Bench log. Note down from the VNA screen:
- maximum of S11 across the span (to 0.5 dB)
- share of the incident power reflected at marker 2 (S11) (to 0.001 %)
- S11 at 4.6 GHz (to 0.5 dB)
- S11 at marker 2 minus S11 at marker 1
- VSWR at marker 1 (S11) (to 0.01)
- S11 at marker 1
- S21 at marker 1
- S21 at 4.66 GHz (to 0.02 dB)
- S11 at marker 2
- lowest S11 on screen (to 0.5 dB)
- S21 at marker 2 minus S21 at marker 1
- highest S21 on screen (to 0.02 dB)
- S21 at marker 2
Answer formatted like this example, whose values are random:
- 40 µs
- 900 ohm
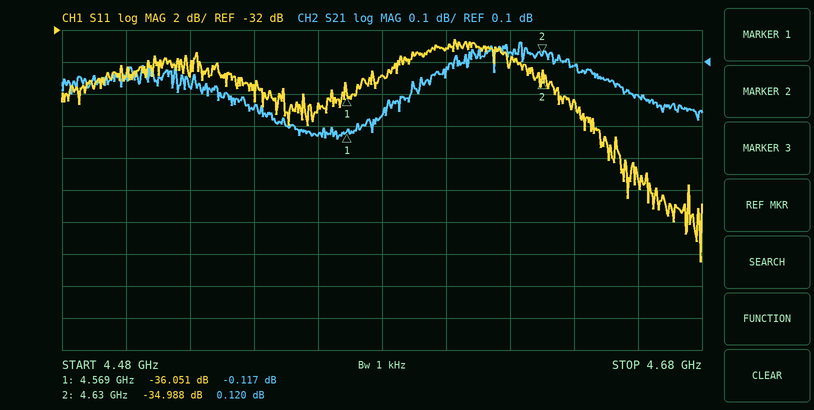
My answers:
- -32.5 dB
- 0.032 %
- -33.0 dB
- 1.063 dB
- 1.03
- -36.051 dB
- -0.117 dB
- 0.00 dB
- -34.988 dB
- -46.5 dB
- 0.237 dB
- 0.16 dB
- 0.120 dB
